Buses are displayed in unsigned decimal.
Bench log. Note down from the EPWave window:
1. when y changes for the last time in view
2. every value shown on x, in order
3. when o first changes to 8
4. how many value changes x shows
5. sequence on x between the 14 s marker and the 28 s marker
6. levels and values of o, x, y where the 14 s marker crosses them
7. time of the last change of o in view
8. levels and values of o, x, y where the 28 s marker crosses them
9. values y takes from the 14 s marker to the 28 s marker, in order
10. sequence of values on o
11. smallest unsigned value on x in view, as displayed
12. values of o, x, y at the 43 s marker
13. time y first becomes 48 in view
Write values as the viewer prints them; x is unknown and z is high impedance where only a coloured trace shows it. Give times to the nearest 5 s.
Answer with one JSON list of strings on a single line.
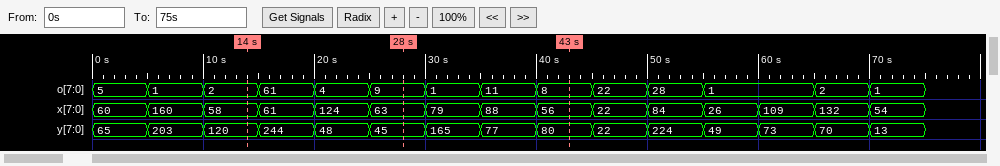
["70 s", "60, 160, 58, 61, 124, 63, 79, 88, 56, 22, 84, 26, 109, 132, 54", "40 s", "14", "58, 61, 124, 63", "o=2, x=58, y=120", "70 s", "o=9, x=63, y=45", "120, 244, 48, 45", "5, 1, 2, 61, 4, 9, 1, 11, 8, 22, 28, 1, 2, 1", "22", "o=8, x=56, y=80", "20 s"]
